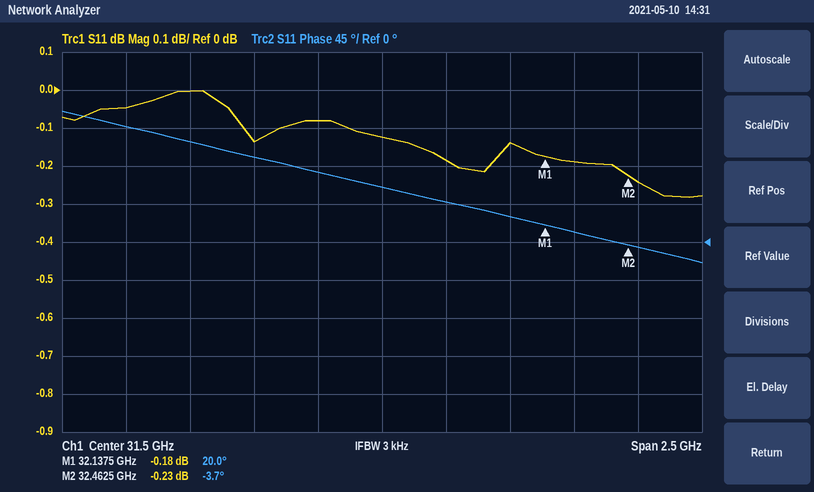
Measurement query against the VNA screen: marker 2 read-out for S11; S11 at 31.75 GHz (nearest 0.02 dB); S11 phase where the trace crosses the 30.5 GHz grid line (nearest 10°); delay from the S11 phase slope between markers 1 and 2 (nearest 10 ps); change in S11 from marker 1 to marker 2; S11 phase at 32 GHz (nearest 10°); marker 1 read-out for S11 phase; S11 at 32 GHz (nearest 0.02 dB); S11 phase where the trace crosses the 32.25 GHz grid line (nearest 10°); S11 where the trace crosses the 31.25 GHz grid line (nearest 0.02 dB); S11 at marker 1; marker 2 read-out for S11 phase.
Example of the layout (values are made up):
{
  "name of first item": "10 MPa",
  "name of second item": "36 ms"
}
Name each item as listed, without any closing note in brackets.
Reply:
{
  "marker 2 read-out for S11": "-0.23 dB",
  "S11 at 31.75 GHz": "-0.18 dB",
  "S11 phase where the trace crosses the 30.5 GHz grid line": "140°",
  "delay from the S11 phase slope between markers 1 and 2": "200 ps",
  "change in S11 from marker 1 to marker 2": "-0.05 dB",
  "S11 phase at 32 GHz": "30°",
  "marker 1 read-out for S11 phase": "20.0°",
  "S11 at 32 GHz": "-0.14 dB",
  "S11 phase where the trace crosses the 32.25 GHz grid line": "10°",
  "S11 where the trace crosses the 31.25 GHz grid line": "-0.08 dB",
  "S11 at marker 1": "-0.18 dB",
  "marker 2 read-out for S11 phase": "-3.7°"
}
